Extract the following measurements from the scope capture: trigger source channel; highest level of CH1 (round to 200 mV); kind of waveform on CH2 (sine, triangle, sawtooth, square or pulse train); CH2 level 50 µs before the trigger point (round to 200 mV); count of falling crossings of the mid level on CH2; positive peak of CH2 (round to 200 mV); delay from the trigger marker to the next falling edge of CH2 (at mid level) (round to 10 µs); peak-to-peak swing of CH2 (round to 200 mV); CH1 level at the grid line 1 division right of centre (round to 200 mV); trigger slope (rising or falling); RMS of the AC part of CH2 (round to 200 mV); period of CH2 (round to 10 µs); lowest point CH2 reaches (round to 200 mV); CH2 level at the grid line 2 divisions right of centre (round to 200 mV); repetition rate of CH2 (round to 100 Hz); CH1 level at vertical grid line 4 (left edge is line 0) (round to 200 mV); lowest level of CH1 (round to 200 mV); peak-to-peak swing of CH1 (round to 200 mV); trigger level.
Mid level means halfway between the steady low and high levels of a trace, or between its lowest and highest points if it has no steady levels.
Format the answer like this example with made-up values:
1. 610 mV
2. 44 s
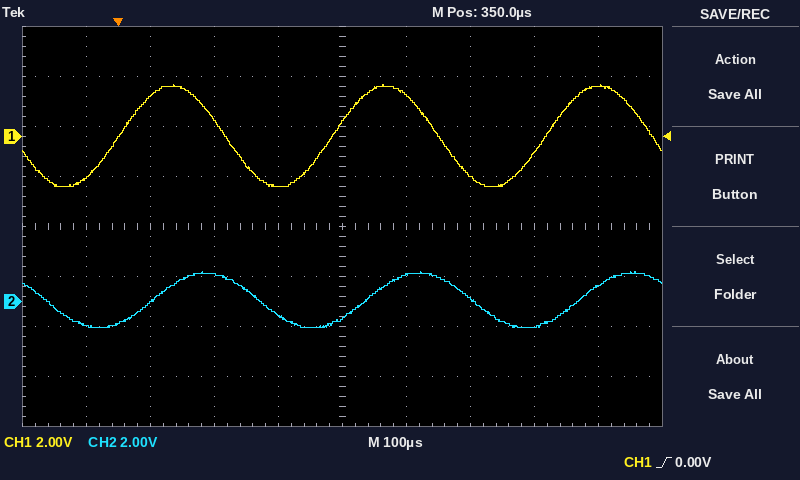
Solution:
1. CH1
2. 2.0 V
3. sine
4. -1.0 V
5. 3
6. 1.2 V
7. 220 µs
8. 2.2 V
9. 1.6 V
10. rising
11. 800 mV
12. 330 µs
13. -1.0 V
14. 200 mV
15. 3.0 kHz
16. -2.0 V
17. -2.0 V
18. 4.0 V
19. 0.00 V
